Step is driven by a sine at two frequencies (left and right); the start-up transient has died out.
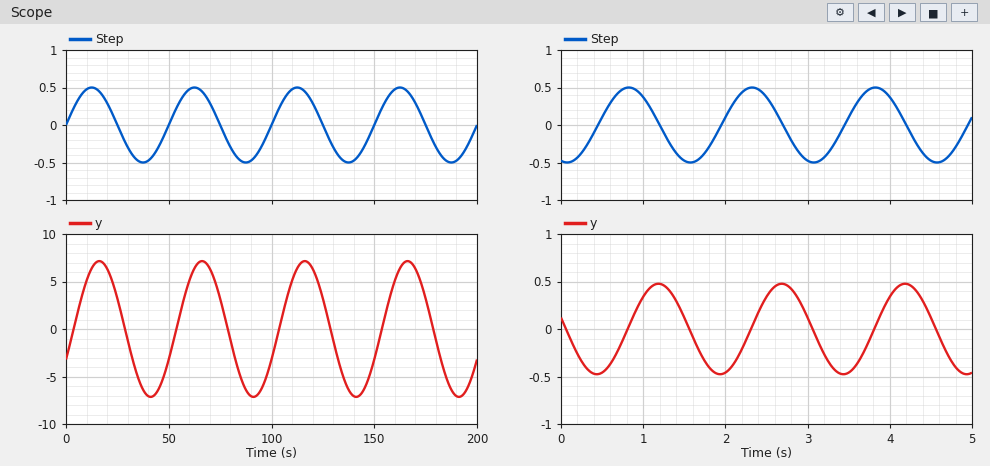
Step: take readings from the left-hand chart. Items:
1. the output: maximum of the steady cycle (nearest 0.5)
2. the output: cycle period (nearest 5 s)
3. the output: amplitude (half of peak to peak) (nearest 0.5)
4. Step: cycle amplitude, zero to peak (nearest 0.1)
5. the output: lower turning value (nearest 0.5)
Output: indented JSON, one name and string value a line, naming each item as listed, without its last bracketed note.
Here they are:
{
  "the output: maximum of the steady cycle": "7.0",
  "the output: cycle period": "50 s",
  "the output: amplitude (half of peak to peak)": "7.0",
  "Step: cycle amplitude, zero to peak": "0.5",
  "the output: lower turning value": "-7.0"
}
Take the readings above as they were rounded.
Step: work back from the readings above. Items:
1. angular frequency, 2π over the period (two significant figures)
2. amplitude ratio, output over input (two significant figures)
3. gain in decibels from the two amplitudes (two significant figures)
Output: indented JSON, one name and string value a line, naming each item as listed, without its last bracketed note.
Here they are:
{
  "angular frequency, 2π over the period": "0.13 rad/s",
  "amplitude ratio, output over input": "14",
  "gain in decibels from the two amplitudes": "23 dB"
}
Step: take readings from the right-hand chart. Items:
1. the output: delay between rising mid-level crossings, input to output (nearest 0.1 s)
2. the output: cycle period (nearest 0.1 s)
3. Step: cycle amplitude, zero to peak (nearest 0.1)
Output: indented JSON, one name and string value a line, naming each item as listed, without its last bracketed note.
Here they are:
{
  "the output: delay between rising mid-level crossings, input to output": "0.4 s",
  "the output: cycle period": "1.5 s",
  "Step: cycle amplitude, zero to peak": "0.5"
}
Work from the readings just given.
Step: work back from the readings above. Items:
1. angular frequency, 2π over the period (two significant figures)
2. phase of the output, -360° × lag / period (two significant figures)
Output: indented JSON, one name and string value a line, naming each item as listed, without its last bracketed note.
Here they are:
{
  "angular frequency, 2π over the period": "4.2 rad/s",
  "phase of the output, -360° × lag / period": "-96°"
}
